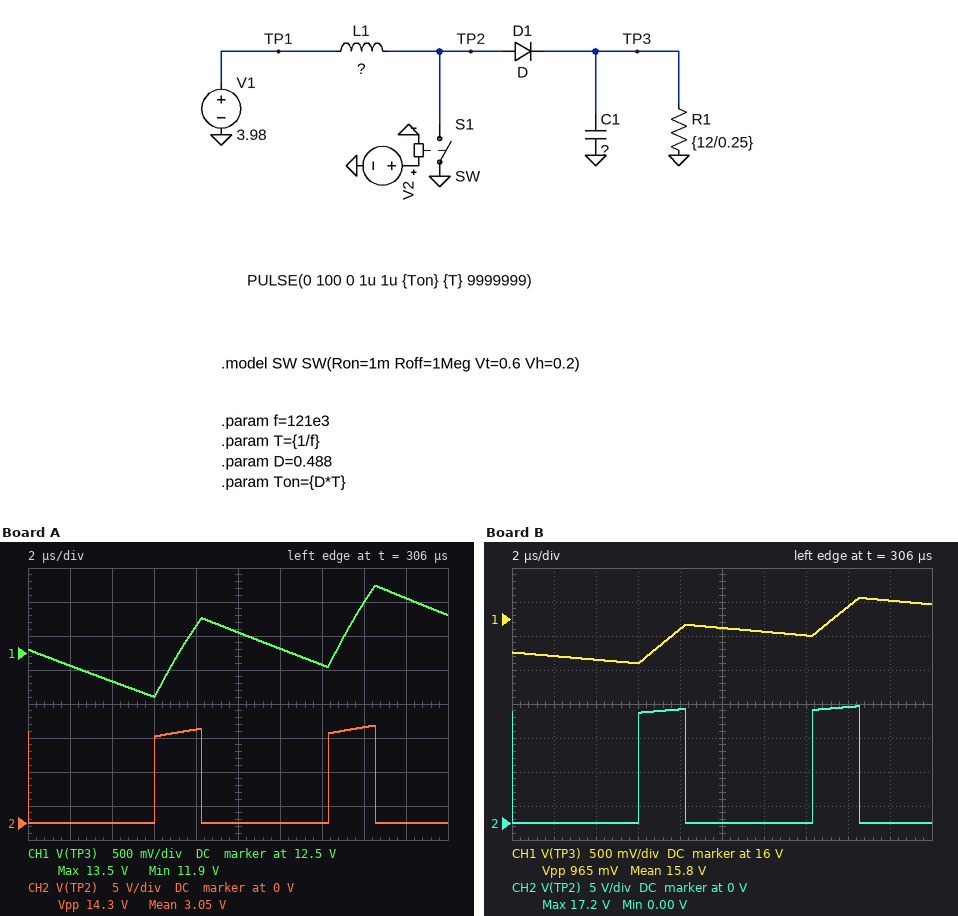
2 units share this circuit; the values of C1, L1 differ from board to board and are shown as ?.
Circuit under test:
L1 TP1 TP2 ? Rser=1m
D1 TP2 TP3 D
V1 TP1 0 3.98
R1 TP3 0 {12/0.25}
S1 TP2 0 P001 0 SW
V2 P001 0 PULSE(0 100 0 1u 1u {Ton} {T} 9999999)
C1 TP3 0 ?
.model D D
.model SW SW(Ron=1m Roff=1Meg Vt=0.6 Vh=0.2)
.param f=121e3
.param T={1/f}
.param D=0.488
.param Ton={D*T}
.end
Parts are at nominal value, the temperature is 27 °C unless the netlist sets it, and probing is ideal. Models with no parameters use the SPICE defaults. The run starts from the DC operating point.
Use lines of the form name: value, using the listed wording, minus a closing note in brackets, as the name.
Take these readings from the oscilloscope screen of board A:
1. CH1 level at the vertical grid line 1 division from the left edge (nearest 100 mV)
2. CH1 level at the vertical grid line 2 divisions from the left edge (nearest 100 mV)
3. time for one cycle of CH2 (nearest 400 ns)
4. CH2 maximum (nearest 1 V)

CH1 level at the vertical grid line 1 division from the left edge: 12.3 V
CH1 level at the vertical grid line 2 divisions from the left edge: 12.1 V
time for one cycle of CH2: 8.4 µs
CH2 maximum: 14 V
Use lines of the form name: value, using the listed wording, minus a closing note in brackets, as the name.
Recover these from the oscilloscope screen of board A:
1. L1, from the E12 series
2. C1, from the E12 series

L1, from the E12 series: 56 µH
C1, from the E12 series: 2.2 µF
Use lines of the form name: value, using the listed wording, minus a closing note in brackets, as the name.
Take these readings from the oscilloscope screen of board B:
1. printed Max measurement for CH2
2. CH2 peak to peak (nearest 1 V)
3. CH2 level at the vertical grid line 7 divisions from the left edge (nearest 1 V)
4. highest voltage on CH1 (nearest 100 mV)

printed Max measurement for CH2: 17.2 V
CH2 peak to peak: 17 V
CH2 level at the vertical grid line 7 divisions from the left edge: 0 V
highest voltage on CH1: 16.3 V
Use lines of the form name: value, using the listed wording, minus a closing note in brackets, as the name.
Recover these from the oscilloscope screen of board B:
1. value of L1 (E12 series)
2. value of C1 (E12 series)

value of L1: 150 µH
value of C1: 12 µF
